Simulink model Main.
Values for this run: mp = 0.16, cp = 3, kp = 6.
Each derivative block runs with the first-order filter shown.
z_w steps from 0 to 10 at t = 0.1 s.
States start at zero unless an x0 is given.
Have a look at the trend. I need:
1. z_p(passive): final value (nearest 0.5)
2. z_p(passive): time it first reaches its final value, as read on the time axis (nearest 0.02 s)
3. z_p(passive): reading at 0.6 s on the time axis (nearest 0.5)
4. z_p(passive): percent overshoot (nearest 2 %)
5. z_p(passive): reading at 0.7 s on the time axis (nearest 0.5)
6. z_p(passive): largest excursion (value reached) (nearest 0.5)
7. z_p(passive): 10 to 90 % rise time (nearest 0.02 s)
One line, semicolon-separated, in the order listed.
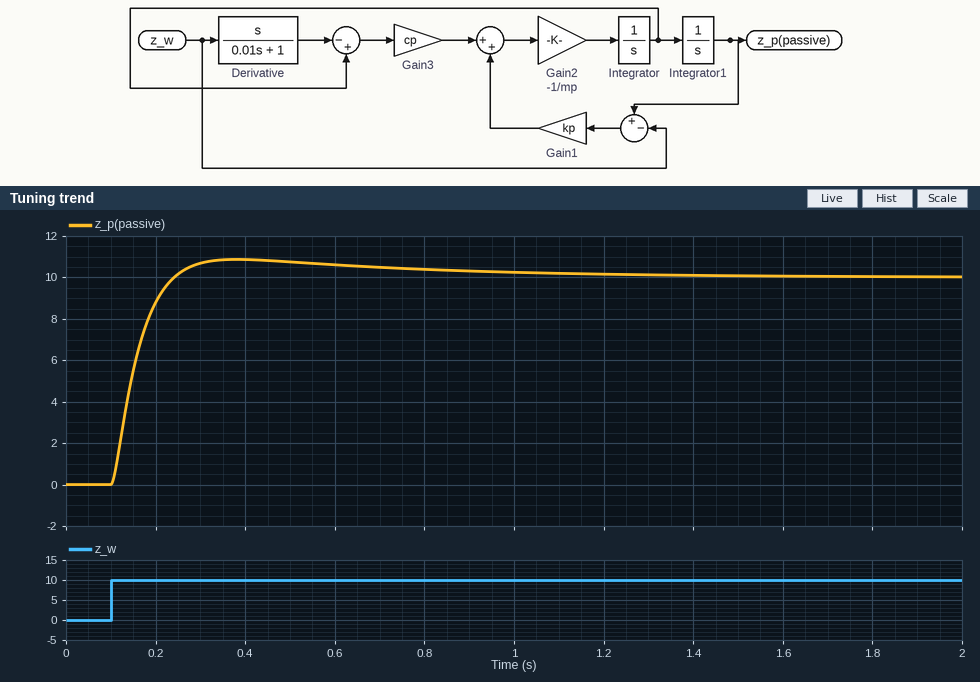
10.0; 0.24 s; 10.5; 8 %; 10.5; 11.0; 0.10 s
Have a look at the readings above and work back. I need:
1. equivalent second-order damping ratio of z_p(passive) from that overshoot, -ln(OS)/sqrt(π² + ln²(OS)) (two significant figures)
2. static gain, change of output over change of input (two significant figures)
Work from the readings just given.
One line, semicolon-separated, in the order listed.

0.63; 1.0
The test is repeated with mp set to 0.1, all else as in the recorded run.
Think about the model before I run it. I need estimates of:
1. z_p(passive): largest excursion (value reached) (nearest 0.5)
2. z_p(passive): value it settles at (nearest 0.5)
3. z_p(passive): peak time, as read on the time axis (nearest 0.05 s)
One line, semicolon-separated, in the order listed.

10.5; 10.0; 0.30 s
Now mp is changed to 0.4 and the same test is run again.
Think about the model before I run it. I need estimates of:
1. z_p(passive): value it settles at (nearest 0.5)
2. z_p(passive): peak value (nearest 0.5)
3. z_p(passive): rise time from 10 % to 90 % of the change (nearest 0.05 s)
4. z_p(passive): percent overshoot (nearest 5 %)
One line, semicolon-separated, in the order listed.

10.0; 11.5; 0.20 s; 15 %
